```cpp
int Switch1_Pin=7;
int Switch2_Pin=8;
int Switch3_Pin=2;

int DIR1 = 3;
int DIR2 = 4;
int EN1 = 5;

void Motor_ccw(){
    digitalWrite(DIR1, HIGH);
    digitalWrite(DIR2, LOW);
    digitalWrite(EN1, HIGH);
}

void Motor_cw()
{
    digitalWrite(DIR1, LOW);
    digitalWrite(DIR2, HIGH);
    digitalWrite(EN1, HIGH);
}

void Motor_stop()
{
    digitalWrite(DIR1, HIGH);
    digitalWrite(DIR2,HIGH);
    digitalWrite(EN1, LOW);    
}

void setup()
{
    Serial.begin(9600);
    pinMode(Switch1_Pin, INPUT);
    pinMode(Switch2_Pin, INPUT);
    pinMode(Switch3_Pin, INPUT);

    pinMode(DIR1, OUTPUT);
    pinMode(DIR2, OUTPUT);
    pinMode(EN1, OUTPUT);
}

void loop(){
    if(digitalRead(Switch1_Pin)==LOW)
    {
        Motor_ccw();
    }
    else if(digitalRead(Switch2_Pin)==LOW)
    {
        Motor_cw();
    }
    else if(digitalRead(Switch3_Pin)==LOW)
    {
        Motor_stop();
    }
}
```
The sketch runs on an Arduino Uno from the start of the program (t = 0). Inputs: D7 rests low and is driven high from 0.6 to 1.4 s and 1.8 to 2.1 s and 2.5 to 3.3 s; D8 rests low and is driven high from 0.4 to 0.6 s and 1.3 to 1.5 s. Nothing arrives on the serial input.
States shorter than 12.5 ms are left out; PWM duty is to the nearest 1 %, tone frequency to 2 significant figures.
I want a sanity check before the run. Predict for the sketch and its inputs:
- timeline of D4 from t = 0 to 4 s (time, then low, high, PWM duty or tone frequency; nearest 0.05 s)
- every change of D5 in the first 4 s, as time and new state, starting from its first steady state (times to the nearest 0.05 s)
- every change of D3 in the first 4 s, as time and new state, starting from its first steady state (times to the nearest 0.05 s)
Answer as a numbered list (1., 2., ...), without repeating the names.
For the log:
1. 0 s low; 0.6 s high; 1.4 s low; 1.8 s high; 2.1 s low; 2.5 s high; 3.3 s low
2. 0 s high; 1.3 s low; 1.4 s high
3. 0 s high; 0.6 s low; 1.3 s high; 1.8 s low; 2.1 s high; 2.5 s low; 3.3 s high
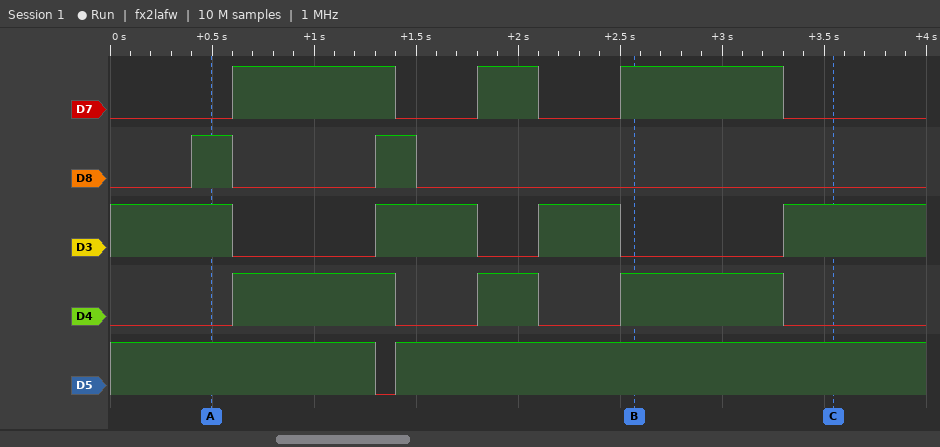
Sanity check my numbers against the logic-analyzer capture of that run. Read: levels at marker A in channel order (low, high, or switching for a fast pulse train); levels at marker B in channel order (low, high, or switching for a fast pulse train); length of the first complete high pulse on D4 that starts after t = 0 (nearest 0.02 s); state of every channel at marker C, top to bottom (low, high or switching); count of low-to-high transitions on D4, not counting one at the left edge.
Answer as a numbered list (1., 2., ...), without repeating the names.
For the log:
1. D7 low, D8 high, D3 high, D4 low, D5 high
2. D7 high, D8 low, D3 low, D4 high, D5 high
3. 0.80 s
4. D7 low, D8 low, D3 high, D4 low, D5 high
5. 3
